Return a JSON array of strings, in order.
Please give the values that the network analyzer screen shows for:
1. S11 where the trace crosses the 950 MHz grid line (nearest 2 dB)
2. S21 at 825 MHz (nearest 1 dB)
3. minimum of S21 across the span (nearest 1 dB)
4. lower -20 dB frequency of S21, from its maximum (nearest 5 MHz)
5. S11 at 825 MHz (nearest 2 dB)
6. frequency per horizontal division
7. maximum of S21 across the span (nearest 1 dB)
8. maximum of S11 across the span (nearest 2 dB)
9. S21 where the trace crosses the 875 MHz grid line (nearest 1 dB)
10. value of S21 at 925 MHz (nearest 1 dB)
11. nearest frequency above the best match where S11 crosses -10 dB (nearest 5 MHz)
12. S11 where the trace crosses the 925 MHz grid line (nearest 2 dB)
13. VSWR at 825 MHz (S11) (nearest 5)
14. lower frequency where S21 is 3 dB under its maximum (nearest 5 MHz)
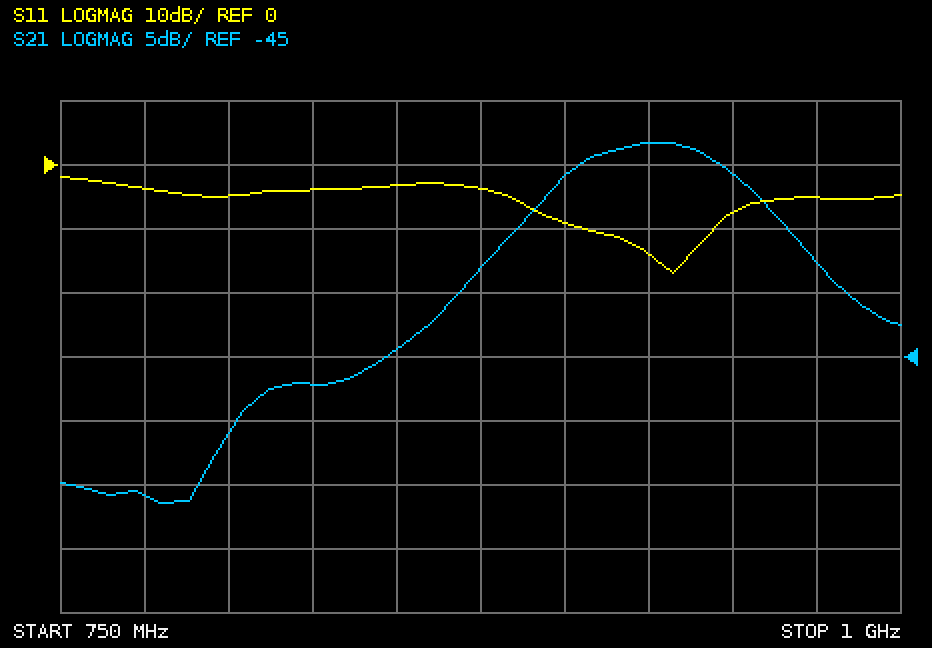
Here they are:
["-8 dB", "-47 dB", "-56 dB", "810 MHz", "-4 dB", "25 MHz", "-28 dB", "-2 dB", "-38 dB", "-28 dB", "945 MHz", "-14 dB", "5", "900 MHz"]
